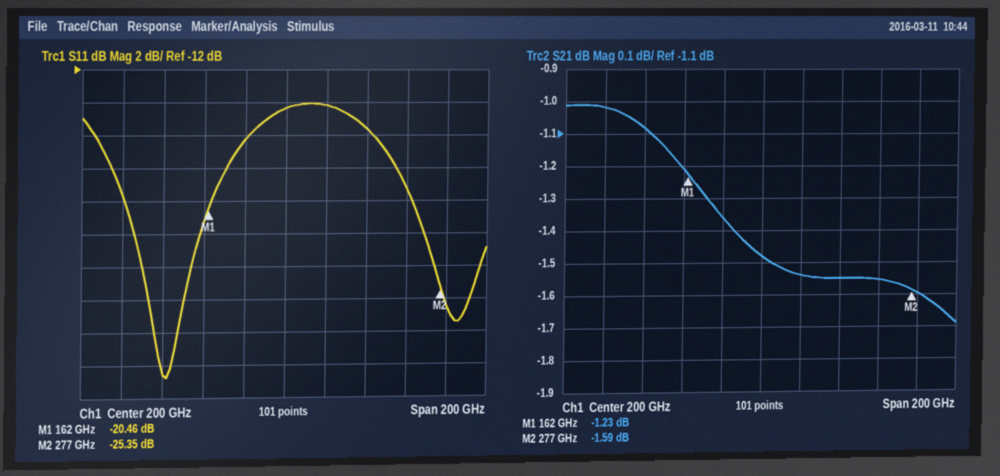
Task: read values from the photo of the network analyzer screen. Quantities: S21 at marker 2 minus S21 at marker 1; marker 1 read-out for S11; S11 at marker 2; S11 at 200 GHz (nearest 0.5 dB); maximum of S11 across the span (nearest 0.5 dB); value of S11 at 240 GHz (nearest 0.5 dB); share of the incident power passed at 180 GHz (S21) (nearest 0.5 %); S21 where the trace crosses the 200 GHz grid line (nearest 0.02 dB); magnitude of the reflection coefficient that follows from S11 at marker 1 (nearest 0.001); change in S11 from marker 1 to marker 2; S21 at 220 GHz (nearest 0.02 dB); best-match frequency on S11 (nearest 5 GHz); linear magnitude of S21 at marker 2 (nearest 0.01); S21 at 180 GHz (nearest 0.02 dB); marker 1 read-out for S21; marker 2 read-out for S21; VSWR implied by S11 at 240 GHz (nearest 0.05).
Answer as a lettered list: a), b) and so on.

a) -0.36 dB
b) -20.46 dB
c) -25.35 dB
d) -14.5 dB
e) -14.0 dB
f) -15.5 dB
g) 73.0 %
h) -1.48 dB
i) 0.095
j) -4.89 dB
k) -1.54 dB
l) 140 GHz
m) 0.83
n) -1.36 dB
o) -1.23 dB
p) -1.59 dB
q) 1.40
